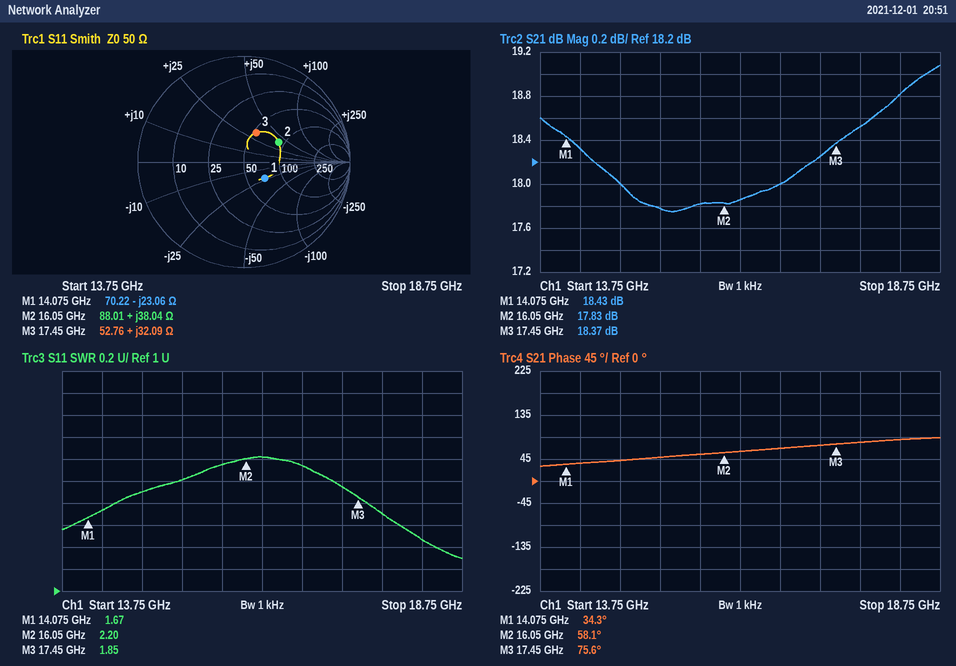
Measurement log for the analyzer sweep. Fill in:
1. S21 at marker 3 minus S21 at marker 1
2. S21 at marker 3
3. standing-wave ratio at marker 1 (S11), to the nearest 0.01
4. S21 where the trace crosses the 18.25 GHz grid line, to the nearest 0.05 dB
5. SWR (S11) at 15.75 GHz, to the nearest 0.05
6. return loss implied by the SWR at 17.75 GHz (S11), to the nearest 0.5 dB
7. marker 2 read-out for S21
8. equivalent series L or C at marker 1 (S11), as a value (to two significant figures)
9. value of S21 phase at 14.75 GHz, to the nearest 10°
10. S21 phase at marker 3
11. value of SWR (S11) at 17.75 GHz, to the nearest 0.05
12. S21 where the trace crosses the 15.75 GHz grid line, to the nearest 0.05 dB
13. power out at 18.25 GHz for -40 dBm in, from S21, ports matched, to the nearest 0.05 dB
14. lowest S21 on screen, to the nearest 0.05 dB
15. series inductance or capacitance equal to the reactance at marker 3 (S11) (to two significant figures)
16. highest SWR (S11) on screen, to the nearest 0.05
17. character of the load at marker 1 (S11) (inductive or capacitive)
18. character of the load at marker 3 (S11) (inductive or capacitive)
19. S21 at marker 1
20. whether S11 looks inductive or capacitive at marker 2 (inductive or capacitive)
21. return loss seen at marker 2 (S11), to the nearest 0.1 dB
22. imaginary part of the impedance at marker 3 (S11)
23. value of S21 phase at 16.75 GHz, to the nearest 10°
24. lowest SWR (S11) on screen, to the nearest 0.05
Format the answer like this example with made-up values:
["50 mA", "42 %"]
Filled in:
["-0.06 dB", "18.37 dB", "1.67", "18.80 dB", "2.15", "11.5 dB", "17.83 dB", "490 fF", "40°", "75.6°", "1.70", "17.80 dB", "-21.20 dBm", "17.75 dB", "290 pH", "2.20", "capacitive", "inductive", "18.43 dB", "inductive", "8.5 dB", "+32.09 Ω", "70°", "1.30"]
